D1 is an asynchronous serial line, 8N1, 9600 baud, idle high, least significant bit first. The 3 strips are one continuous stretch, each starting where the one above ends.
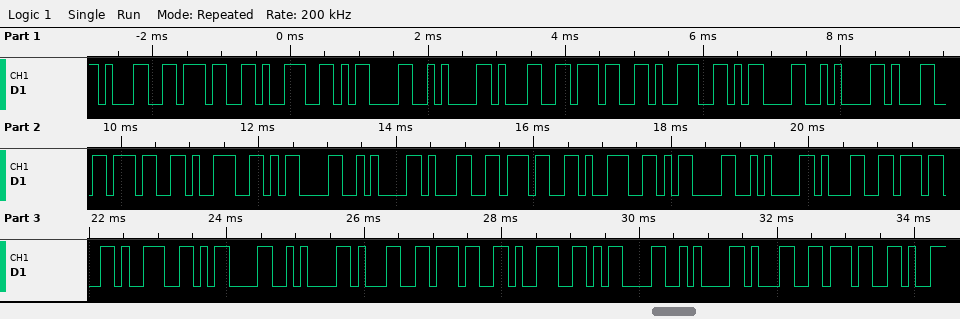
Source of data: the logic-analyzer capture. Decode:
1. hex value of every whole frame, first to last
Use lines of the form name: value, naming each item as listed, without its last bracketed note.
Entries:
hex value of every whole frame, first to last: 31 37 39 0D 0A 31 37 39 0D 0A 31 37 39 0D 0A 31 37 39 0D 0A 31 37 39 0D 0A 31 37 39 0D 0A 31 37
